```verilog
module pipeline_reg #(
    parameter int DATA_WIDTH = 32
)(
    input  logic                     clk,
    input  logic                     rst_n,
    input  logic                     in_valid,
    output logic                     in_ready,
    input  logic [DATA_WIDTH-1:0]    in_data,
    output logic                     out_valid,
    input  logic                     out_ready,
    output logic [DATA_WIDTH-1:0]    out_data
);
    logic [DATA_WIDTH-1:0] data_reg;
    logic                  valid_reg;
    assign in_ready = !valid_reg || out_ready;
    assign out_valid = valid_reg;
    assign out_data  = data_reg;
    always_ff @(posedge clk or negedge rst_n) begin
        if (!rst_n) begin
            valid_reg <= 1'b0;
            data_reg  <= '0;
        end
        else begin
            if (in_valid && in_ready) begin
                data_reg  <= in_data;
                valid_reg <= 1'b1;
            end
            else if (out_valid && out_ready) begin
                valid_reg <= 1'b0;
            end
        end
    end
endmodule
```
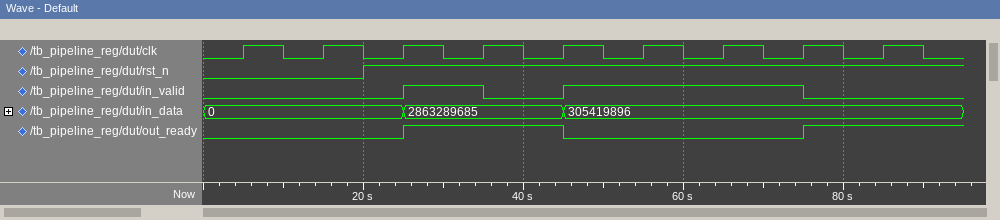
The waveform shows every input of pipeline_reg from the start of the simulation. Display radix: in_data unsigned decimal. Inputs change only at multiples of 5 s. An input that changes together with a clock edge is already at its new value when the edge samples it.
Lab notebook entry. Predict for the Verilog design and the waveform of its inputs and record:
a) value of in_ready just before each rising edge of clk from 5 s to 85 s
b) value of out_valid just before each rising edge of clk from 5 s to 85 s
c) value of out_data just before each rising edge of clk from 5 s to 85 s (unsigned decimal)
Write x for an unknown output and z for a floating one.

1 1 1 1 1 0 0 0 1
0 0 0 1 0 1 1 1 0
0, 0, 0, 2863289685, 2863289685, 305419896, 305419896, 305419896, 305419896
